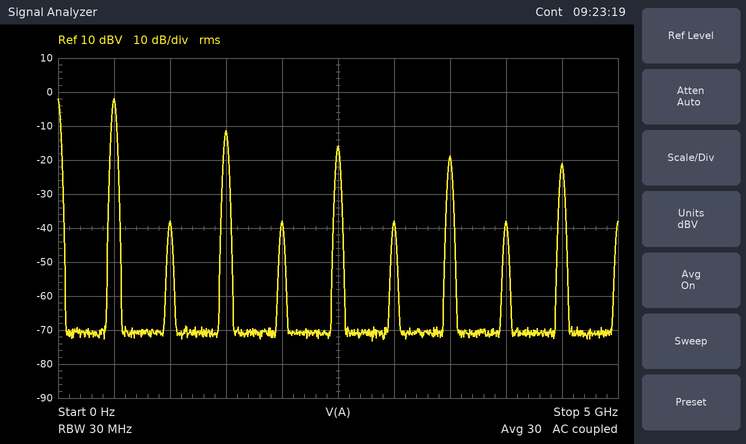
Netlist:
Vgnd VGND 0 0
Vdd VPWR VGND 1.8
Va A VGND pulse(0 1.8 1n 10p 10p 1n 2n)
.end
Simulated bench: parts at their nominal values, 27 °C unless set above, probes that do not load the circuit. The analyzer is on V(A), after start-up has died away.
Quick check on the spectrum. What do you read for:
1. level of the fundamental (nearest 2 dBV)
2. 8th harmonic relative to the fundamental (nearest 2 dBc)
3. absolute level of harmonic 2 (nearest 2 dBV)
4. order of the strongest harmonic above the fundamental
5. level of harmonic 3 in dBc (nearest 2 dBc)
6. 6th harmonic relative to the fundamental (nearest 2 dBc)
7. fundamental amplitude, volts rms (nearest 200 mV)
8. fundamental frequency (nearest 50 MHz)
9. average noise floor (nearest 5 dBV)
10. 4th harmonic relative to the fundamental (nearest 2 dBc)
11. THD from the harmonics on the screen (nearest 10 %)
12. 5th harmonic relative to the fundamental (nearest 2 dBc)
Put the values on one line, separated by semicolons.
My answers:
-2 dBV; -36 dBc; -38 dBV; 3; -10 dBc; -36 dBc; 800 mV; 500 MHz; -70 dBV; -36 dBc; 40 %; -14 dBc
